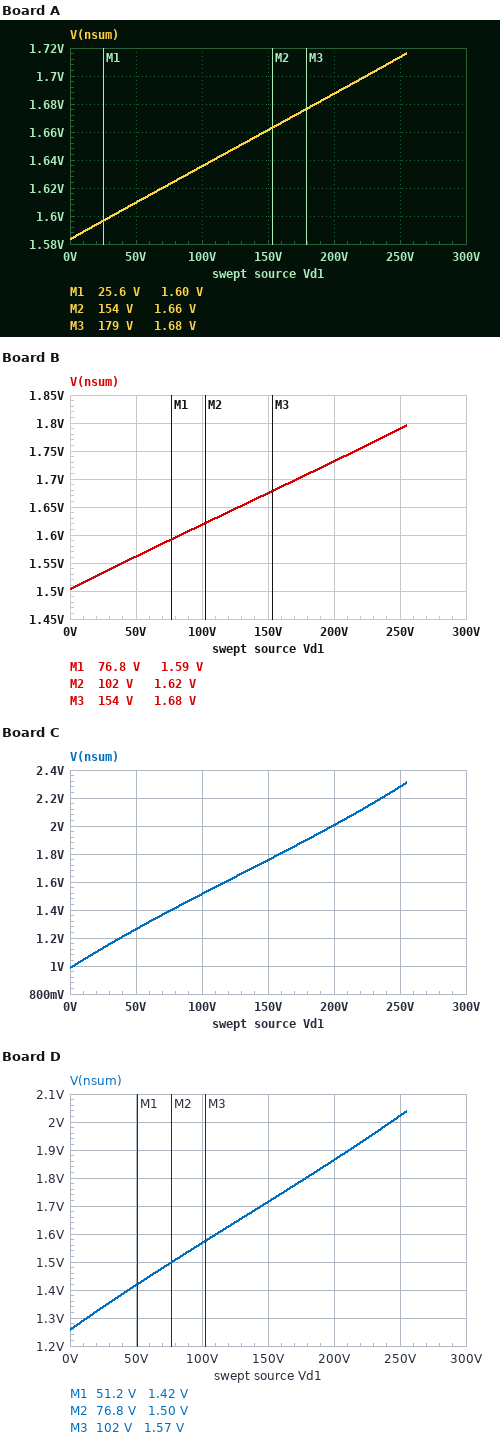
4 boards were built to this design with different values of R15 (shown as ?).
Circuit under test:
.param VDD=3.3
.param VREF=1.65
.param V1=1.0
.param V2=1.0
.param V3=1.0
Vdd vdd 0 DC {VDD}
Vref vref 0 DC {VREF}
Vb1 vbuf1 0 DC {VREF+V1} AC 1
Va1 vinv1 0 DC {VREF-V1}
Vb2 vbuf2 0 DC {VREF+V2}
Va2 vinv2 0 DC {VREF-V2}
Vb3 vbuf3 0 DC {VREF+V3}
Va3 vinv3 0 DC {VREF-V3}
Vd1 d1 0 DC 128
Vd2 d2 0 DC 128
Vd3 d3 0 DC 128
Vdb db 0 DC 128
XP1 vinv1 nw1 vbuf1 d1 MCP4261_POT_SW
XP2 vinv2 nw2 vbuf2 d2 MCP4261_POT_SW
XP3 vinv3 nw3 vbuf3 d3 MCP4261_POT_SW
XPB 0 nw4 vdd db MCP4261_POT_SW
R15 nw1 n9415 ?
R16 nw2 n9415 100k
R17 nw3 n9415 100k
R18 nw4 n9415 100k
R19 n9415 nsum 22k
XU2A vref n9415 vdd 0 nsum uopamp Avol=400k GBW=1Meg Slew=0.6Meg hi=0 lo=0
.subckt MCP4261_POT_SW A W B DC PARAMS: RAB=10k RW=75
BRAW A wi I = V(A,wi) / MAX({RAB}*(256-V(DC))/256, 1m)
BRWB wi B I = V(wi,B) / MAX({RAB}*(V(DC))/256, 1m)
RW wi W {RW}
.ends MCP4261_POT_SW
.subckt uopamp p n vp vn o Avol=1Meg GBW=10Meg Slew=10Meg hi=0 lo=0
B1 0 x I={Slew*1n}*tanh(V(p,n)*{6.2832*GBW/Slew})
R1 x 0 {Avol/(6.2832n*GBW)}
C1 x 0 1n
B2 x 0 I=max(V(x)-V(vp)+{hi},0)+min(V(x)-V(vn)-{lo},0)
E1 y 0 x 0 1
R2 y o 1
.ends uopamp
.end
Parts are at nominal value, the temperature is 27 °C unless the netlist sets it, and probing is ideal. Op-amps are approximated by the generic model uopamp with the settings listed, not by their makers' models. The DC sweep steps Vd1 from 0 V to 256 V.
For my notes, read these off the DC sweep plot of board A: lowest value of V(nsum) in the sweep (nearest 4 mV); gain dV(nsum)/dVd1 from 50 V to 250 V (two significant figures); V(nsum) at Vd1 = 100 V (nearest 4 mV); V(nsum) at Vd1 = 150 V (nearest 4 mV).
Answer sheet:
1.584 V
0.00052 V/V
1.636 V
1.660 V
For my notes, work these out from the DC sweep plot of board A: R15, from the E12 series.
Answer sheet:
330 kΩ
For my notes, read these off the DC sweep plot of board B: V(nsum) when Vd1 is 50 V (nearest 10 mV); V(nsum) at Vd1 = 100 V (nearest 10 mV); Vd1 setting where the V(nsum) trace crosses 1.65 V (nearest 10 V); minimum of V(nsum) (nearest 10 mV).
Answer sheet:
1.56 V
1.62 V
130 V
1.50 V
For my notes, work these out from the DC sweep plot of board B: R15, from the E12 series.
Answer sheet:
150 kΩ
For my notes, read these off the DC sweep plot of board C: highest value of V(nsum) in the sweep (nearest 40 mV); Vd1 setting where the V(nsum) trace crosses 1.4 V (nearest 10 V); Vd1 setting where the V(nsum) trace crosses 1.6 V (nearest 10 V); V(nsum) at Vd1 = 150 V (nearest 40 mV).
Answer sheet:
2.32 V
80 V
120 V
1.76 V
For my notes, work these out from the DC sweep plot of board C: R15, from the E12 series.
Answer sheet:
33 kΩ
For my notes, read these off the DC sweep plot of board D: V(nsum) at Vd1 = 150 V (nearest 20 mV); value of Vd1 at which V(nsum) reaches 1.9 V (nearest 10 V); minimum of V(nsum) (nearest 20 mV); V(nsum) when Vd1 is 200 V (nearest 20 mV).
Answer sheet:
1.72 V
210 V
1.26 V
1.86 V
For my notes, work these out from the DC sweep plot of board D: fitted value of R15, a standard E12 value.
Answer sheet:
56 kΩ
